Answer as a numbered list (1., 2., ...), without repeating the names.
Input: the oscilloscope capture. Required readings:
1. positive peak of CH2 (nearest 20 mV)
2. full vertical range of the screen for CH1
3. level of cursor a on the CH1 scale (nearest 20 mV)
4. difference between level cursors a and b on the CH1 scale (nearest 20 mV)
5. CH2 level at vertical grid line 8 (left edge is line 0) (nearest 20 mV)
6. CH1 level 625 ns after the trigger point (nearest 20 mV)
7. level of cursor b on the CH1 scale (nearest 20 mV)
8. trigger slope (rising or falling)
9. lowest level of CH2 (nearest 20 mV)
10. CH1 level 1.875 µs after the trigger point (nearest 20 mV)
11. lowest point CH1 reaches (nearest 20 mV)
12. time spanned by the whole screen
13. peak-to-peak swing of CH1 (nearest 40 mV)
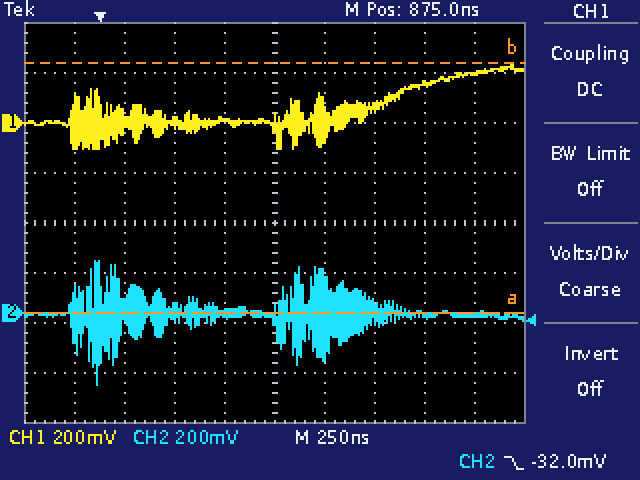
1. 200 mV
2. 1.6 V
3. -760 mV
4. 1.00 V
5. 0 mV
6. 20 mV
7. 240 mV
8. falling
9. -280 mV
10. 200 mV
11. -100 mV
12. 2.5 µs
13. 320 mV
